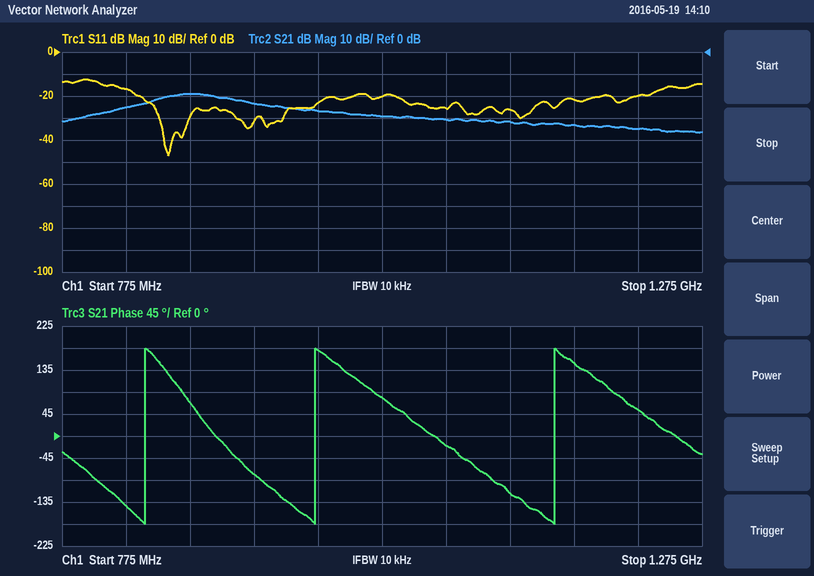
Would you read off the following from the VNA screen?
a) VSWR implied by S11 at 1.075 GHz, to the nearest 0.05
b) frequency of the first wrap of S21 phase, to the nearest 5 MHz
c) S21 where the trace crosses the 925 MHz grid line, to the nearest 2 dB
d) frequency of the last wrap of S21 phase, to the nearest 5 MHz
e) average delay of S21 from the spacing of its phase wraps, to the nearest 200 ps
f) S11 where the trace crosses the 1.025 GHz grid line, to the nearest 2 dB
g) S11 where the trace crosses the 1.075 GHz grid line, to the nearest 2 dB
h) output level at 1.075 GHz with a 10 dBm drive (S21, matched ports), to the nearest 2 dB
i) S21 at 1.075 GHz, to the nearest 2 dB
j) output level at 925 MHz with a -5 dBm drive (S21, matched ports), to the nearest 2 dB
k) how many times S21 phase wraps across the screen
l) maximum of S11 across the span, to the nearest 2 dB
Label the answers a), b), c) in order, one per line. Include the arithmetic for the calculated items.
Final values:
a) |Γ| = 10^(-26/20) = 0.0501; VSWR = (1 + 0.0501)/(1 − 0.0501) ≈ 1.11, so 1.10 to the nearest 0.05
b) 840 MHz
c) -24 dB
d) 1.160 GHz
e) 2 cycles / (1.160 GHz − 840 MHz) ≈ 6.2 ns
f) -20 dB
g) -26 dB
h) 10 dBm + (-30 dB) = -20 dBm
i) -30 dB
j) -5 dBm + (-24 dB) = -28 dBm
k) 3
l) -12 dB
